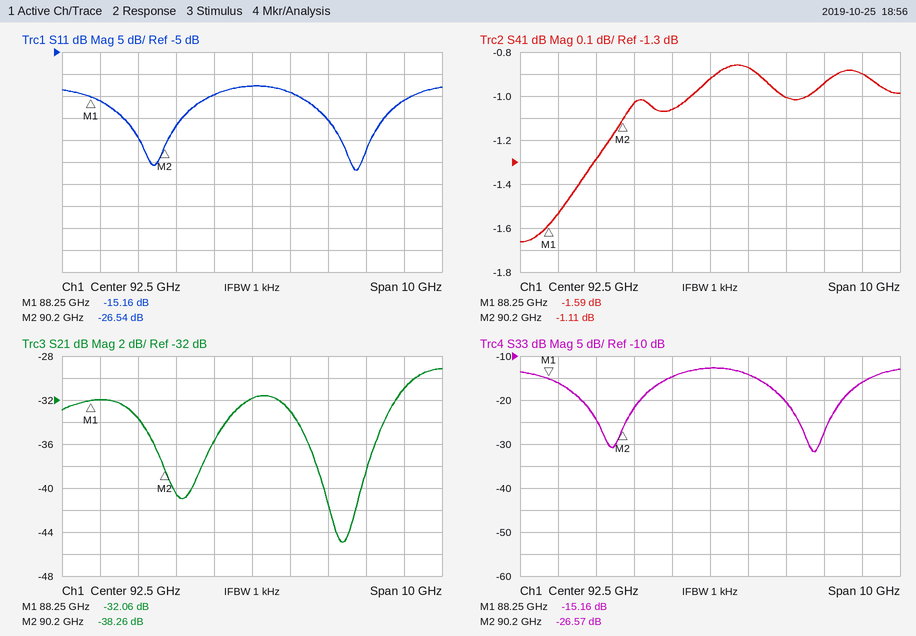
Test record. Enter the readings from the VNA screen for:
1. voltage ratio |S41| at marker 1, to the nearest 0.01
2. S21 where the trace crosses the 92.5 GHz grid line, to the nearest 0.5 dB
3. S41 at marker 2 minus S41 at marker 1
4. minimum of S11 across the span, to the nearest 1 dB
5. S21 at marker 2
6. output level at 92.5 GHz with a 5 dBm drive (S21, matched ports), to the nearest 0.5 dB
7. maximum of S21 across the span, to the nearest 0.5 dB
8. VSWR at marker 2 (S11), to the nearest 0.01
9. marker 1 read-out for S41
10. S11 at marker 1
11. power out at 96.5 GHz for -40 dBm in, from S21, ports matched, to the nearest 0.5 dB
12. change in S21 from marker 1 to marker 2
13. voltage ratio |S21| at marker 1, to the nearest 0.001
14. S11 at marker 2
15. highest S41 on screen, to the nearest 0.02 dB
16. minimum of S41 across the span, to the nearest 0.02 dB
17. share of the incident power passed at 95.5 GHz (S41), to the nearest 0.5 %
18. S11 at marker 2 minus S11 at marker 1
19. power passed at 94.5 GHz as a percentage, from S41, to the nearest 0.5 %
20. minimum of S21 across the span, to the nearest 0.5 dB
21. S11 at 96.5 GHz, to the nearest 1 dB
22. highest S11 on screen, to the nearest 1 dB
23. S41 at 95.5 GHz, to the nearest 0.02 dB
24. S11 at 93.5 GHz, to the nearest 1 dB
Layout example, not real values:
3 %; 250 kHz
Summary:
0.83; -32.0 dB; 0.48 dB; -32 dB; -38.26 dB; -27.0 dBm; -29.0 dB; 1.10; -1.59 dB; -15.16 dB; -71.0 dBm; -6.20 dB; 0.025; -26.54 dB; -0.86 dB; -1.66 dB; 80.5 %; -11.38 dB; 79.5 %; -45.0 dB; -16 dB; -13 dB; -0.94 dB; -14 dB
